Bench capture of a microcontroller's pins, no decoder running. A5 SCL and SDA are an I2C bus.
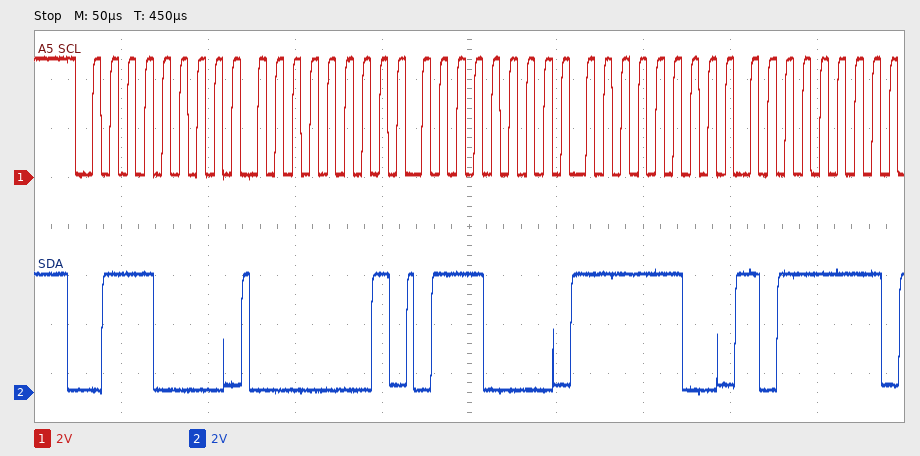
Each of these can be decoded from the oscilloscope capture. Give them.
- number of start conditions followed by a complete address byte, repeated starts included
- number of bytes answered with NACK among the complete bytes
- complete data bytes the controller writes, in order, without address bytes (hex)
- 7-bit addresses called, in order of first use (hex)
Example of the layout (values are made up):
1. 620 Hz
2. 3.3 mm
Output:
1. 1
2. 0
3. 01 70 FC BF
4. 0x38
